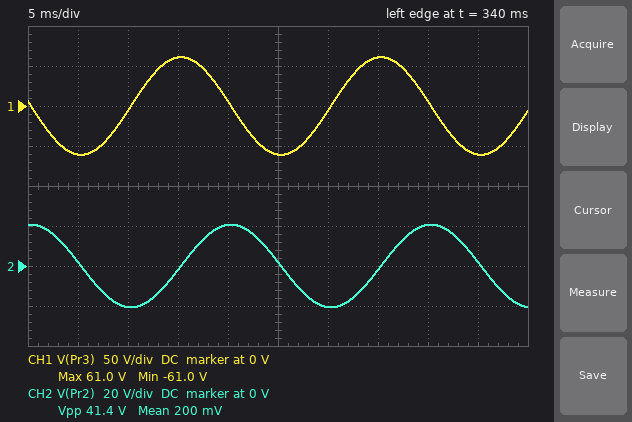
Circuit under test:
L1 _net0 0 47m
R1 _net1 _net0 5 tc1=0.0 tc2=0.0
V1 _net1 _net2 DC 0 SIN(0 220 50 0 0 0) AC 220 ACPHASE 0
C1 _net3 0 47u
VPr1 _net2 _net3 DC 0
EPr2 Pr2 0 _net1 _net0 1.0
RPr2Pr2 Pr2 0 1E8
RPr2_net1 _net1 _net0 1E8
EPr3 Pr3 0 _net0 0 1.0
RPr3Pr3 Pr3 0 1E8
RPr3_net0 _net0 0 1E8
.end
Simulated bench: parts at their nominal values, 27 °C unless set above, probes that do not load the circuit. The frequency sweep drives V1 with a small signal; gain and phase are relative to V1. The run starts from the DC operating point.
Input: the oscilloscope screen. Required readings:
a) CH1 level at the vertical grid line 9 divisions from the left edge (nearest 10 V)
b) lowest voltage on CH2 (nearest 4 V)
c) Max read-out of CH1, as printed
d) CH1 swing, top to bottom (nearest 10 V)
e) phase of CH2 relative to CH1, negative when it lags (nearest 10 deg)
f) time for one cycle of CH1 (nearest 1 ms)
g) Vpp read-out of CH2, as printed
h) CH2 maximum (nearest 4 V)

-60 V
-20 V
61.0 V
120 V
-90 deg
20 ms
41.4 V
20 V
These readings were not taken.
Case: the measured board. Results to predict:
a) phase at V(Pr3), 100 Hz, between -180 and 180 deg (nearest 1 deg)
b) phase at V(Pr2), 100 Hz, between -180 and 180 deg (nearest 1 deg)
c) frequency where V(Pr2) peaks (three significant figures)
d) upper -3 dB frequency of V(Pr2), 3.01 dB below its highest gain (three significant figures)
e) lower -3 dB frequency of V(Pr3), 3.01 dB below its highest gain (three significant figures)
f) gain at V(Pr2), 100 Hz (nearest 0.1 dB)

131 deg
41 deg
107 Hz
116 Hz
100 Hz
-2.4 dB
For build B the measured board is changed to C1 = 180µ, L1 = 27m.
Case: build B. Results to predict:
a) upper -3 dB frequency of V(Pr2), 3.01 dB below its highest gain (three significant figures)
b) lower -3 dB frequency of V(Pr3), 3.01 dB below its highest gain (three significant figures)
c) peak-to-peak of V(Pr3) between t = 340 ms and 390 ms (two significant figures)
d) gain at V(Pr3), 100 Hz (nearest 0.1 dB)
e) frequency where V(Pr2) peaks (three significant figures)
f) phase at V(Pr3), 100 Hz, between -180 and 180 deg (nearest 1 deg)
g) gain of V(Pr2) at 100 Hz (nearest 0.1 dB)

88.4 Hz
62.9 Hz
360 V
5.0 dB
72.2 Hz
32 deg
-5.6 dB
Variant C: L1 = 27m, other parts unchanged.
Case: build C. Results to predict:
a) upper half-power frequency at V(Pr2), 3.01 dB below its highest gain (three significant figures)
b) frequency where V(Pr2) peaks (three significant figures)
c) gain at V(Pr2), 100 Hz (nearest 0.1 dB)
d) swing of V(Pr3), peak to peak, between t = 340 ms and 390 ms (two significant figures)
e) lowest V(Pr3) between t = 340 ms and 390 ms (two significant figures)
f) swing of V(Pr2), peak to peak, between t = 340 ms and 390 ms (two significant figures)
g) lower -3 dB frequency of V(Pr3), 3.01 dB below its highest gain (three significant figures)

157 Hz
141 Hz
-10.9 dB
63 V
-31 V
37 V
130 Hz
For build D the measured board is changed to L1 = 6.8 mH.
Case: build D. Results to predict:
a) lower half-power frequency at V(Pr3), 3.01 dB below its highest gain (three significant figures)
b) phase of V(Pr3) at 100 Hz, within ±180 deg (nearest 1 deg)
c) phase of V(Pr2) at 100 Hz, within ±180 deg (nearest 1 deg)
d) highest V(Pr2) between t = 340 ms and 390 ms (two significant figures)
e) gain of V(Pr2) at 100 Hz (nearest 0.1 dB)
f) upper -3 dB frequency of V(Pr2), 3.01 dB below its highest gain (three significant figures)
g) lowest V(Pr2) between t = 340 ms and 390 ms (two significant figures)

245 Hz
170 deg
80 deg
17 V
-15.6 dB
346 Hz
-17 V
